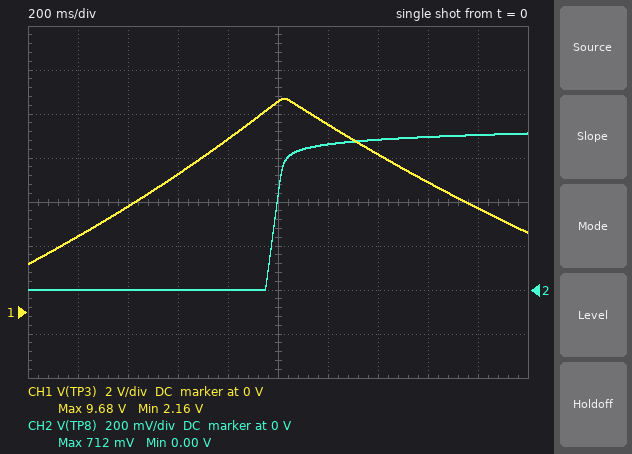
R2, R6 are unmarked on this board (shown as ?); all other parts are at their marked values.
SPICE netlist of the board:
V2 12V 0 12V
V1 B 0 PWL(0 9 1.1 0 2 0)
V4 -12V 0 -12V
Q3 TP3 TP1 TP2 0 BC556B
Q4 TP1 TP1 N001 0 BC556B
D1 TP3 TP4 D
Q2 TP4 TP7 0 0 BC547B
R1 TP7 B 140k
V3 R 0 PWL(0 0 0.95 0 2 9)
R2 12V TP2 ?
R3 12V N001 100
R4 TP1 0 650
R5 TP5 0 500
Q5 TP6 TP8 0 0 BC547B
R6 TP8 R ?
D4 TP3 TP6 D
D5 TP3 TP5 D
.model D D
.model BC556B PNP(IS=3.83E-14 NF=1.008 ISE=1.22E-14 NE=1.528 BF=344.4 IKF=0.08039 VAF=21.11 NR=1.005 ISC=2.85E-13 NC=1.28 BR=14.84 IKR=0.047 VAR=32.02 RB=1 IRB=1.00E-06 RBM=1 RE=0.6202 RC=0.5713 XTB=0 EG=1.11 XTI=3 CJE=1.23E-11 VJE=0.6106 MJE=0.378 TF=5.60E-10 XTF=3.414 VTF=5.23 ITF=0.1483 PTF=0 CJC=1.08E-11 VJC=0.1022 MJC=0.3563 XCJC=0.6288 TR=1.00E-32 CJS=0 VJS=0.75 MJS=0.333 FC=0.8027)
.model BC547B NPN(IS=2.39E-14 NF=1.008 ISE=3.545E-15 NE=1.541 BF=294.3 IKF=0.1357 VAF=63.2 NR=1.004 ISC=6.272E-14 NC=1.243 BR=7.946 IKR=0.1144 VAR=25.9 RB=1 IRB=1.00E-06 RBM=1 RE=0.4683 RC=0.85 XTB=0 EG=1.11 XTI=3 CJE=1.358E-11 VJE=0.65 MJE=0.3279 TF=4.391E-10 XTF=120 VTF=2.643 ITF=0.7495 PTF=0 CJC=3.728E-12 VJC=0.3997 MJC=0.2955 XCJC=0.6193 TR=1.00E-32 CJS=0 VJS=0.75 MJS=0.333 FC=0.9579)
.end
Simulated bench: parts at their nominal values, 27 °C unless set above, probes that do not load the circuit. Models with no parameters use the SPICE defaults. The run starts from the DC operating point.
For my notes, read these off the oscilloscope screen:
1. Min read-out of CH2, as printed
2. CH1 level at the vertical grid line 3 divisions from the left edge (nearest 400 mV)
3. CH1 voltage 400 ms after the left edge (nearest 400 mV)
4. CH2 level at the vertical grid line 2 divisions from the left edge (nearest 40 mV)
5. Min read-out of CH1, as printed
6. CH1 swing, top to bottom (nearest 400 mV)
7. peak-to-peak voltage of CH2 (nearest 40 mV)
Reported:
0.00 V
6.4 V
4.8 V
0 V
2.16 V
7.6 V
720 mV
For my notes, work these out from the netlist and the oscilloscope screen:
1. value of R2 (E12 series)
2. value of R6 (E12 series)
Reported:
82 Ω
180 kΩ
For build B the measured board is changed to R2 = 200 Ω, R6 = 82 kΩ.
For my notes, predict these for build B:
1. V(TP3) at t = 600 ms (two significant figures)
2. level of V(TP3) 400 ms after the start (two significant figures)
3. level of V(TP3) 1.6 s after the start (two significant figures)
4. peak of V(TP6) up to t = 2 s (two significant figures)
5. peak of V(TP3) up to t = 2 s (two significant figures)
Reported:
1.2 V
850 mV
820 mV
3.9 V
4.4 V
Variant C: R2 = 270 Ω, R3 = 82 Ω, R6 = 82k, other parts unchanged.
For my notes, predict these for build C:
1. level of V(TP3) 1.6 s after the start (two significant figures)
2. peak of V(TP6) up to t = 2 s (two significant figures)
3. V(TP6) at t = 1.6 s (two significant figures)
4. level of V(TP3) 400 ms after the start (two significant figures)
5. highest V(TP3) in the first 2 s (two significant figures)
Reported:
780 mV
2.5 V
86 mV
800 mV
3.0 V
